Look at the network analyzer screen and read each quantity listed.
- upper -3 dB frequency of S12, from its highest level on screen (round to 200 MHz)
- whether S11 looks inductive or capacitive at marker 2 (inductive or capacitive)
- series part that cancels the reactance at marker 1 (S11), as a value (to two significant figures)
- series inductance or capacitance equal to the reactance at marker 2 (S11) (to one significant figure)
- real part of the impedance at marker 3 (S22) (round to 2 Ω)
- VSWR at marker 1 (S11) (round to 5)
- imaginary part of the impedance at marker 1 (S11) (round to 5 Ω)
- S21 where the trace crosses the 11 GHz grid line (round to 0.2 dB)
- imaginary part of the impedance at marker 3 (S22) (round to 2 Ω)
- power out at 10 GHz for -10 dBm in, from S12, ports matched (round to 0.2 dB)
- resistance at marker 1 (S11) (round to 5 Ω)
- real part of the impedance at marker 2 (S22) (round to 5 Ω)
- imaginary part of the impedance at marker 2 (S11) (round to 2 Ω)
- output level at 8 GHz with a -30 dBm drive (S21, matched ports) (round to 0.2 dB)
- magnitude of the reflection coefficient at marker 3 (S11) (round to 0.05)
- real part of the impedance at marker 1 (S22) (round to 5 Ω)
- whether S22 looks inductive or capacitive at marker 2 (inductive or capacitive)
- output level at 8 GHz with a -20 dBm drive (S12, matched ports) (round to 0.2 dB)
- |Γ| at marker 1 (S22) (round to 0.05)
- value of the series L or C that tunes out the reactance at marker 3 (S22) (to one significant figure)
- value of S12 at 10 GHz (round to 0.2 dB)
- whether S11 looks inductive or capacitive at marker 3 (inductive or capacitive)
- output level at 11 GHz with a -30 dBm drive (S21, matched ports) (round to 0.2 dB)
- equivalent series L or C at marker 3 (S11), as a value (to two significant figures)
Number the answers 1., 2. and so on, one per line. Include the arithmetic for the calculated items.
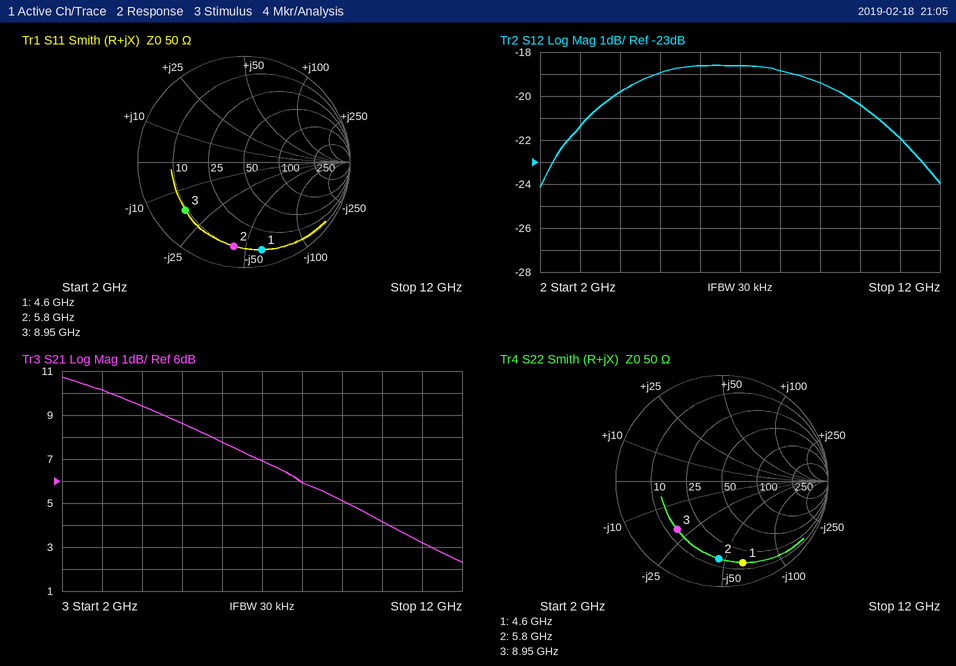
1. 10.8 GHz
2. capacitive
3. L = 60 Ω/(2π × 4.6 GHz) ≈ 2.1 nH
4. C = 1/(2π × 5.8 GHz × 44 Ω) ≈ 624 fF, so 600 fF to one significant figure
5. 14 Ω
6. 10
7. -60 Ω
8. 3.2 dB
9. -20 Ω
10. -10 dBm + (-20.4 dB) = -30.4 dBm
11. 10 Ω
12. 15 Ω
13. -44 Ω
14. -30 dBm + (6.0 dB) = -24.0 dBm
15. 0.70
16. 15 Ω
17. capacitive
18. -20 dBm + (-18.8 dB) = -38.8 dBm
19. 0.80
20. L = 20 Ω/(2π × 8.95 GHz) ≈ 356 pH, so 400 pH to one significant figure
21. -20.4 dB
22. capacitive
23. -30 dBm + (3.2 dB) = -26.8 dBm
24. C = 1/(2π × 8.95 GHz × 18 Ω) ≈ 1.0 pF
